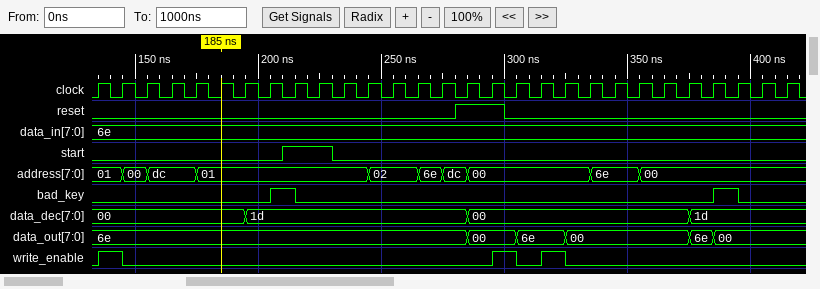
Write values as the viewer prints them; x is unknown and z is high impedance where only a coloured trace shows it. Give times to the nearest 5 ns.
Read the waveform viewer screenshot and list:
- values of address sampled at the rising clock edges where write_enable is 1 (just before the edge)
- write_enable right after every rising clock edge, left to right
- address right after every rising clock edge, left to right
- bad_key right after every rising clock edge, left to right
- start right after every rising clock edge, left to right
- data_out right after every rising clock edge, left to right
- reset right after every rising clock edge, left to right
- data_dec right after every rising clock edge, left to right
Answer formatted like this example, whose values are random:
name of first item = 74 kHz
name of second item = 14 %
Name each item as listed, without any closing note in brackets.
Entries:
values of address sampled at the rising clock edges where write_enable is 1 = 01, 00, 00
write_enable right after every rising clock edge, left to right = 1 0 0 0 0 0 0 0 0 0 0 0 0 0 0 0 1 0 1 0 0 0 0 0 0 0 0 0 0
address right after every rising clock edge, left to right = 01, 00, dc, dc, 01, 01, 01, 01, 01, 01, 01, 02, 02, 6e, dc, 00, 00, 00, 00, 00, 6e, 6e, 00, 00, 00, 00, 00, 00, 00
bad_key right after every rising clock edge, left to right = 0 0 0 0 0 0 0 1 0 0 0 0 0 0 0 0 0 0 0 0 0 0 0 0 0 1 0 0 0
start right after every rising clock edge, left to right = 0 0 0 0 0 0 0 0 1 1 0 0 0 0 0 0 0 0 0 0 0 0 0 0 0 0 0 0 0
data_out right after every rising clock edge, left to right = 6e, 6e, 6e, 6e, 6e, 6e, 6e, 6e, 6e, 6e, 6e, 6e, 6e, 6e, 6e, 00, 00, 6e, 6e, 00, 00, 00, 00, 00, 6e, 00, 00, 00, 00
reset right after every rising clock edge, left to right = 0 0 0 0 0 0 0 0 0 0 0 0 0 0 0 1 1 0 0 0 0 0 0 0 0 0 0 0 0
data_dec right after every rising clock edge, left to right = 00, 00, 00, 00, 00, 00, 1d, 1d, 1d, 1d, 1d, 1d, 1d, 1d, 1d, 00, 00, 00, 00, 00, 00, 00, 00, 00, 1d, 1d, 1d, 1d, 1d
